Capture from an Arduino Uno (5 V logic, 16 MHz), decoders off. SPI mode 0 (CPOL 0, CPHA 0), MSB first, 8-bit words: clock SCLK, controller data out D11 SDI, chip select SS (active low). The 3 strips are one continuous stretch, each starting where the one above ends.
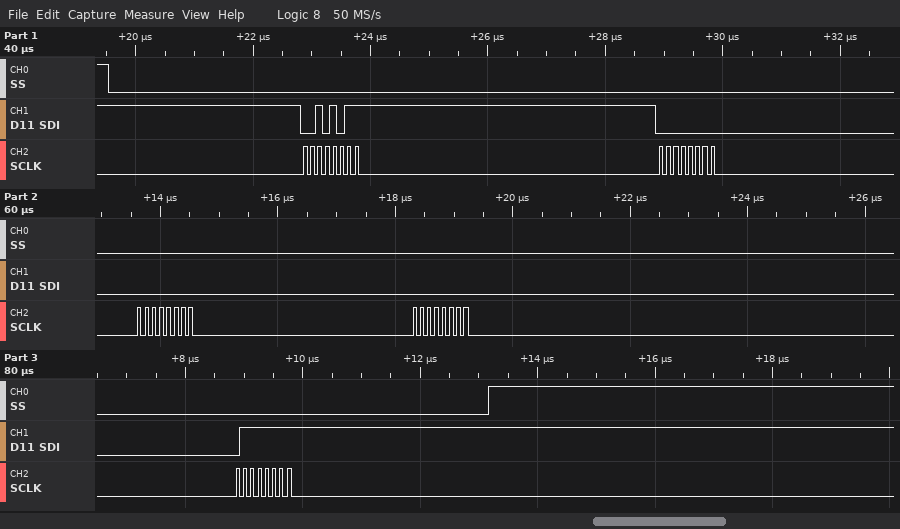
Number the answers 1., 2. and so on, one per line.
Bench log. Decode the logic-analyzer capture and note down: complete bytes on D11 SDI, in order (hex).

1. 2B 00 00 00 7F
